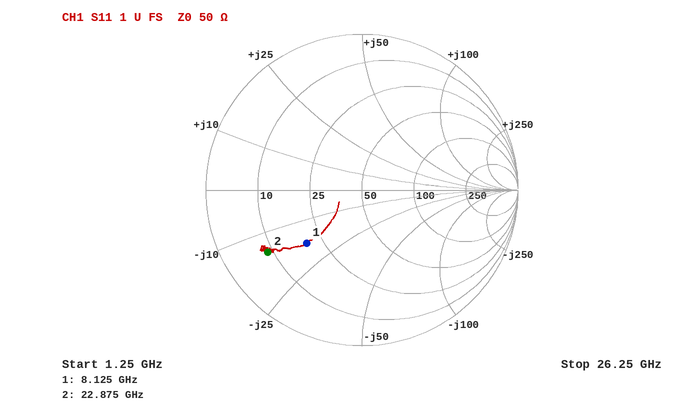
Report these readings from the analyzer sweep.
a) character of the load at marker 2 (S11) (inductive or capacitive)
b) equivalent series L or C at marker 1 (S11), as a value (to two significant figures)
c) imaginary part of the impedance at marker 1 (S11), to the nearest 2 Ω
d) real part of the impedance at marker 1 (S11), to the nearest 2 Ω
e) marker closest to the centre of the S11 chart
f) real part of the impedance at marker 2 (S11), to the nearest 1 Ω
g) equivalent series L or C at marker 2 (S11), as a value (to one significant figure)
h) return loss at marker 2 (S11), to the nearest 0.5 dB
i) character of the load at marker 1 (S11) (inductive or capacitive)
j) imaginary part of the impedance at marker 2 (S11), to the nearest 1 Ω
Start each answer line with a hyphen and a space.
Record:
- capacitive
- 1.1 pF
- -18 Ω
- 20 Ω
- marker 1
- 9 Ω
- 500 fF
- 3.0 dB
- capacitive
- -15 Ω
